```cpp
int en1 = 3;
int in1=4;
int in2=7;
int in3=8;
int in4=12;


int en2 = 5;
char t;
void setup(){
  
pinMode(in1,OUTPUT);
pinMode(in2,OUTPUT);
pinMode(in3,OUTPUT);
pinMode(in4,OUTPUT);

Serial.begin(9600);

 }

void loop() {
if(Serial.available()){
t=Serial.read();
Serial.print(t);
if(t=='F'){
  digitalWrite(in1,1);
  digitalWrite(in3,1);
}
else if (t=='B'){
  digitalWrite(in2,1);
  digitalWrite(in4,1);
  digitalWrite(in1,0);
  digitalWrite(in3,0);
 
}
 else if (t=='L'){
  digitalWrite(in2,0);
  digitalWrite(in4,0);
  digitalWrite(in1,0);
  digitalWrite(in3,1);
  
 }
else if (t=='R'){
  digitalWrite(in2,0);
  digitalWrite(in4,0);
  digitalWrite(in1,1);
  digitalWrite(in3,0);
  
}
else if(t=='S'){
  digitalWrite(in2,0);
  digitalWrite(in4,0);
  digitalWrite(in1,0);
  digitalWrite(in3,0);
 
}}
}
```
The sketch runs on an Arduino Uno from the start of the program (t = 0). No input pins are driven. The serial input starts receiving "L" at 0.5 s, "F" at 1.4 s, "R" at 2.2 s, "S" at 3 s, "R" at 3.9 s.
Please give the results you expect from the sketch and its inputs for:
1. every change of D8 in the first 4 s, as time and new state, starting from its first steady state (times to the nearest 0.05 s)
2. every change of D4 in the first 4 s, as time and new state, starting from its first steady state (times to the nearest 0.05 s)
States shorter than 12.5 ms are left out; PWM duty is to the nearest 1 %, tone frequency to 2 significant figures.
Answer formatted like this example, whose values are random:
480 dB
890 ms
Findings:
0 s low; 0.5 s high; 2.2 s low
0 s low; 1.4 s high; 3 s low; 3.9 s high
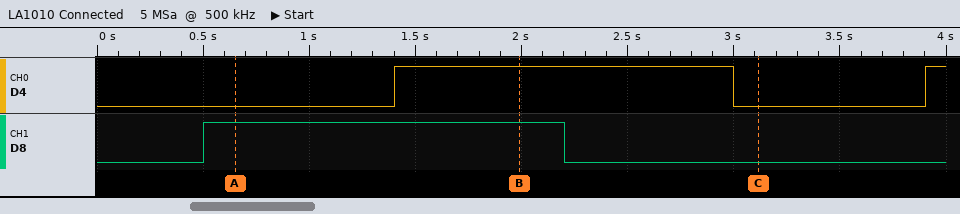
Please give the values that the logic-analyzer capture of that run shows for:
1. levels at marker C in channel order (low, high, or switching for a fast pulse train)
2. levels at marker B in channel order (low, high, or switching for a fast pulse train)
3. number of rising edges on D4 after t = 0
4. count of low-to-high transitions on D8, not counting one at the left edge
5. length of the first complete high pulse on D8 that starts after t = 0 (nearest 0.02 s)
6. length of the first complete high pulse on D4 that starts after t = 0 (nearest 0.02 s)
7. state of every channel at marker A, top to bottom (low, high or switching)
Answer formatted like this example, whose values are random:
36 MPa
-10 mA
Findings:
D4 low, D8 low
D4 high, D8 high
2
1
1.70 s
1.60 s
D4 low, D8 high
